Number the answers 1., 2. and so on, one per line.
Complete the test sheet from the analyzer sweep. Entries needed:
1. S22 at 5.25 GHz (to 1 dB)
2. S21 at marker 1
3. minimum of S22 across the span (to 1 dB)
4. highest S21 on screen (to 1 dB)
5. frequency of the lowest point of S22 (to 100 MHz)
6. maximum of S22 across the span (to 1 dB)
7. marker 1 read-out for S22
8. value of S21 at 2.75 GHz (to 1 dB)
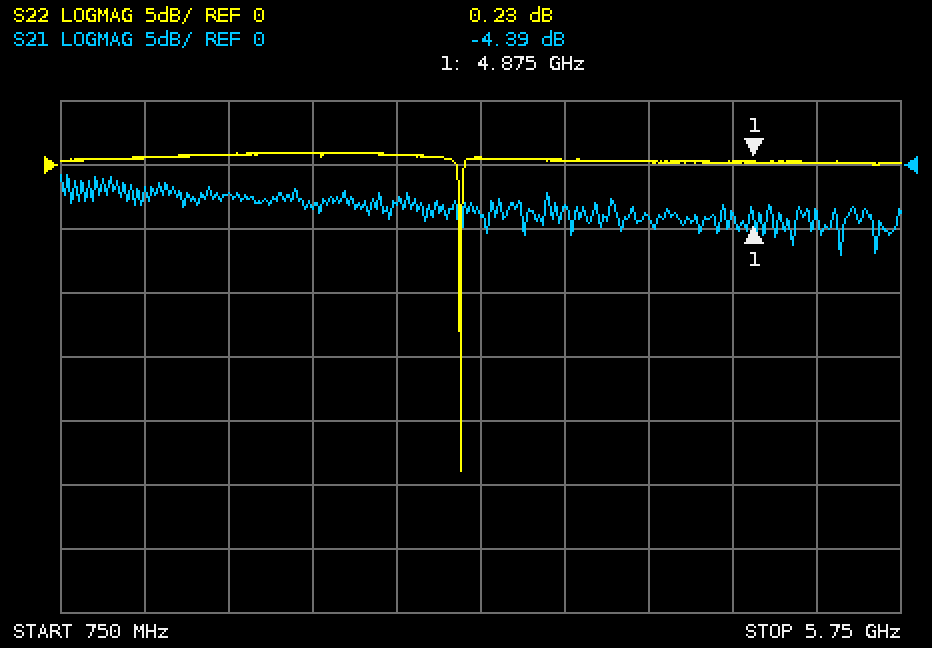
1. 0 dB
2. -4.39 dB
3. -24 dB
4. -1 dB
5. 3.1 GHz
6. 1 dB
7. 0.23 dB
8. -3 dB
